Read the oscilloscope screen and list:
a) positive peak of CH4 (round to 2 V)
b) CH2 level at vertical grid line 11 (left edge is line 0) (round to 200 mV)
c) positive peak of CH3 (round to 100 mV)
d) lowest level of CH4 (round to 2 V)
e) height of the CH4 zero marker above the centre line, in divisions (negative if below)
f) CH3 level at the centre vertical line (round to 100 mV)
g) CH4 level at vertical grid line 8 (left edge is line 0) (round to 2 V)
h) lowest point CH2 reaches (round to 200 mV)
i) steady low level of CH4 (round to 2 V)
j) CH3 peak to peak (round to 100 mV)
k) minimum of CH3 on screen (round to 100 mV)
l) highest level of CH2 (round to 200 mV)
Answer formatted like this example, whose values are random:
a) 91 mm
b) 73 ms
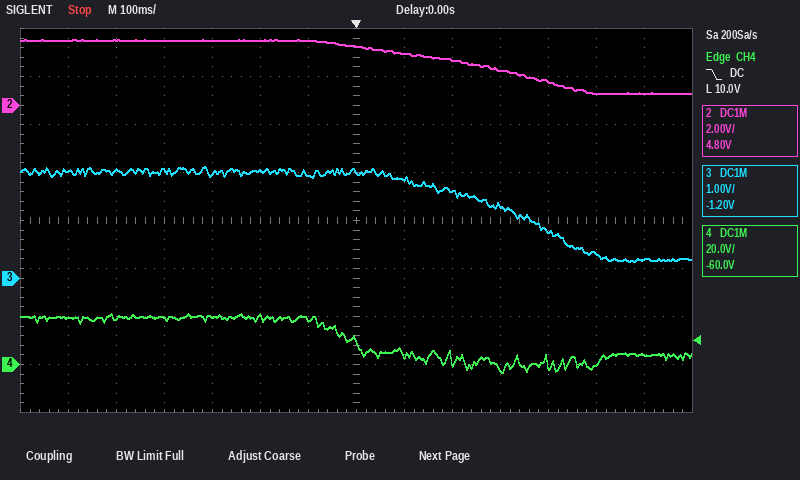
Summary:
a) 22 V
b) 1.0 V
c) 2.3 V
d) -4 V
e) -3.0 div
f) 2.2 V
g) 4 V
h) 400 mV
i) 4 V
j) 2.0 V
k) 300 mV
l) 2.8 V
